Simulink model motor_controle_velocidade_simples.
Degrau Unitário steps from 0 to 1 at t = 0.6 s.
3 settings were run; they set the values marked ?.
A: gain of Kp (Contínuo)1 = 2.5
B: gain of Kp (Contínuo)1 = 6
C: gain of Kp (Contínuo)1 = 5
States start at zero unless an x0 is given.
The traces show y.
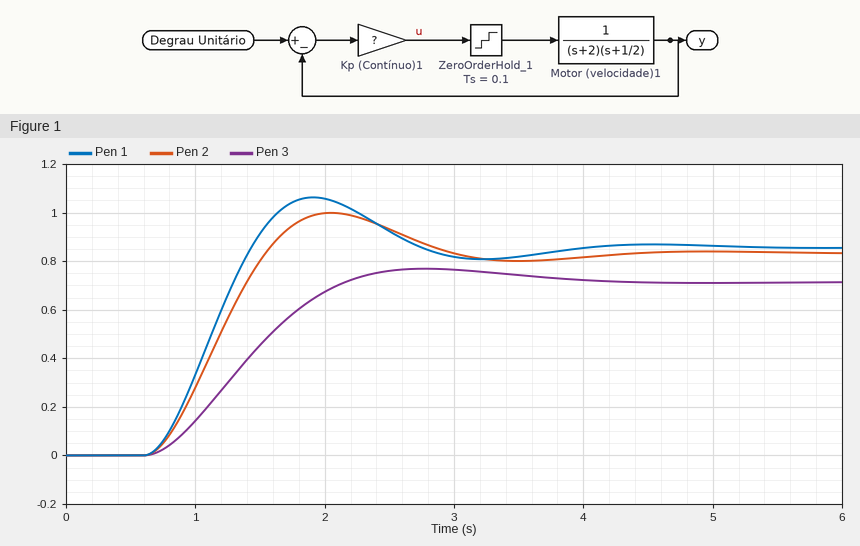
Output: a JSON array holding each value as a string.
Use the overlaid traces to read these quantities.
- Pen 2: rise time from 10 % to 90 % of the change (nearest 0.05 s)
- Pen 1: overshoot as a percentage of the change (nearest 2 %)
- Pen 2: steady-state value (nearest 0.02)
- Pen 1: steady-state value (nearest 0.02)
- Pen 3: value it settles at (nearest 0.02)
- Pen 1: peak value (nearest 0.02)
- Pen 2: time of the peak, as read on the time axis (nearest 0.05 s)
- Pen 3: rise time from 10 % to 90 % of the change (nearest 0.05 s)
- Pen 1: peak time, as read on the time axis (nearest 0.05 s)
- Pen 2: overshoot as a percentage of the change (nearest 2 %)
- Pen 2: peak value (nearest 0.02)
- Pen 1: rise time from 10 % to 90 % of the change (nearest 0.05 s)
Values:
["0.65 s", "24 %", "0.84", "0.86", "0.72", "1.06", "2.05 s", "1.05 s", "1.90 s", "20 %", "1.00", "0.55 s"]
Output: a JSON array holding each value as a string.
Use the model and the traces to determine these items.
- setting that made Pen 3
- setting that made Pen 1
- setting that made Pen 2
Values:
["A", "B", "C"]
